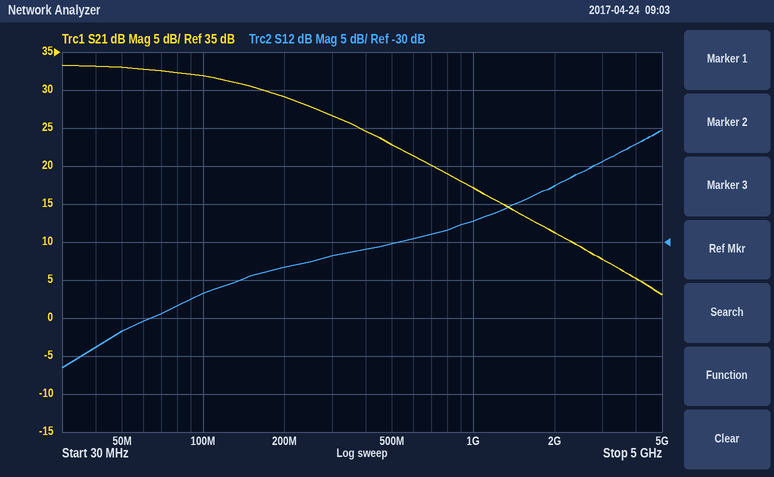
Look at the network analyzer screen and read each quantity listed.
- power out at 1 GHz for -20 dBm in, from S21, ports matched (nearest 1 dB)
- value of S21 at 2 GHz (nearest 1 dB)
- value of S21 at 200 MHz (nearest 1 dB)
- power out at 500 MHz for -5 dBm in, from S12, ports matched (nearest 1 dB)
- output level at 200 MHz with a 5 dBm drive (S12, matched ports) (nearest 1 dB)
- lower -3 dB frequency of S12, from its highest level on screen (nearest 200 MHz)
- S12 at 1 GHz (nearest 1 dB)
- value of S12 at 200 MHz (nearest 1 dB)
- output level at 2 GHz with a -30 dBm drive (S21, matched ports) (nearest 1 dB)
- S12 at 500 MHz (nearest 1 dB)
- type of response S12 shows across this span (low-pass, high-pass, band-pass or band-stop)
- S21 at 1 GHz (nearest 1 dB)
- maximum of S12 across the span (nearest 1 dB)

-3 dBm
11 dB
29 dB
-35 dBm
-28 dBm
3.4 GHz
-27 dB
-33 dB
-19 dBm
-30 dB
high-pass
17 dB
-15 dB
